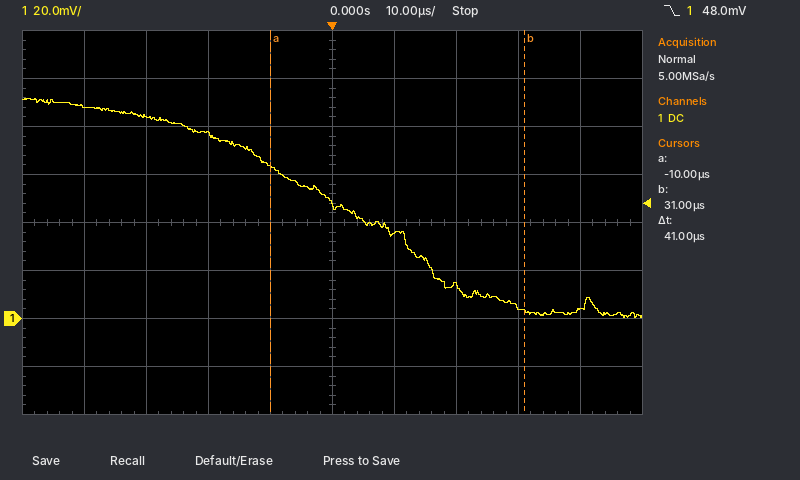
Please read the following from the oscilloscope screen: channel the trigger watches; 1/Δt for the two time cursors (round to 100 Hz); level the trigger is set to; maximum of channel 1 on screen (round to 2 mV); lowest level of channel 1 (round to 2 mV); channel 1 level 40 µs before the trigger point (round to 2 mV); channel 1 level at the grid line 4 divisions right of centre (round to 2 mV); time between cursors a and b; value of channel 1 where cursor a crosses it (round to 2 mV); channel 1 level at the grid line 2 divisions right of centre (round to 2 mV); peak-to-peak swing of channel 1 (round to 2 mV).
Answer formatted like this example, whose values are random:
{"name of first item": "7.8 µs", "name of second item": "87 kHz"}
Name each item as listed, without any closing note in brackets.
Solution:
{"channel the trigger watches": "channel 1", "1/Δt for the two time cursors": "24.4 kHz", "level the trigger is set to": "48.0 mV", "maximum of channel 1 on screen": "92 mV", "lowest level of channel 1": "0 mV", "channel 1 level 40 µs before the trigger point": "88 mV", "channel 1 level at the grid line 4 divisions right of centre": "4 mV", "time between cursors a and b": "41 µs", "value of channel 1 where cursor a crosses it": "64 mV", "channel 1 level at the grid line 2 divisions right of centre": "14 mV", "peak-to-peak swing of channel 1": "92 mV"}
